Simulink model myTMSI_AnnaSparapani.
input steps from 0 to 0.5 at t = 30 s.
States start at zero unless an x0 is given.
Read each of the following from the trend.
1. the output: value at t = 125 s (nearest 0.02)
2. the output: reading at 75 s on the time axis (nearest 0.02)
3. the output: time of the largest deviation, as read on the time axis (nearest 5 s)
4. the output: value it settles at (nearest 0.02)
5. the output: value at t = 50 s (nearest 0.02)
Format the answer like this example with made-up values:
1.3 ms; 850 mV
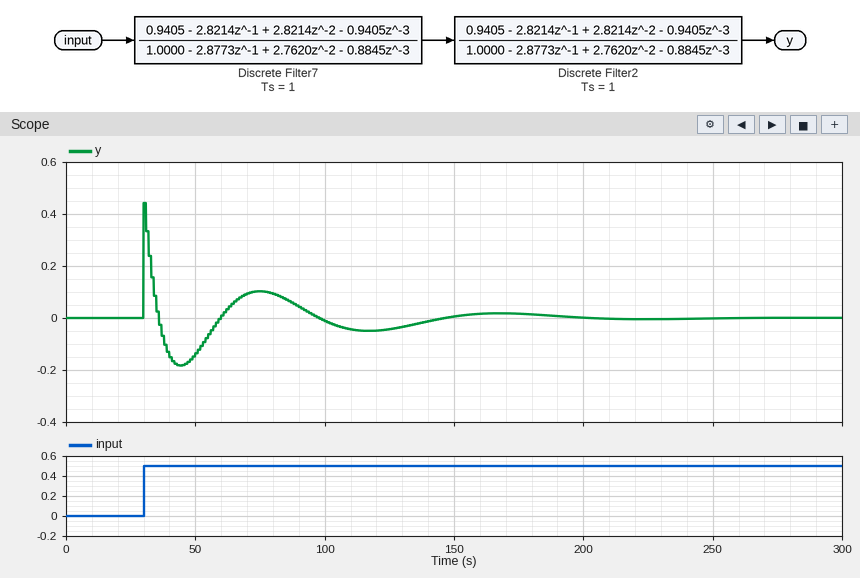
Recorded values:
-0.04; 0.10; 30 s; 0.00; -0.14
